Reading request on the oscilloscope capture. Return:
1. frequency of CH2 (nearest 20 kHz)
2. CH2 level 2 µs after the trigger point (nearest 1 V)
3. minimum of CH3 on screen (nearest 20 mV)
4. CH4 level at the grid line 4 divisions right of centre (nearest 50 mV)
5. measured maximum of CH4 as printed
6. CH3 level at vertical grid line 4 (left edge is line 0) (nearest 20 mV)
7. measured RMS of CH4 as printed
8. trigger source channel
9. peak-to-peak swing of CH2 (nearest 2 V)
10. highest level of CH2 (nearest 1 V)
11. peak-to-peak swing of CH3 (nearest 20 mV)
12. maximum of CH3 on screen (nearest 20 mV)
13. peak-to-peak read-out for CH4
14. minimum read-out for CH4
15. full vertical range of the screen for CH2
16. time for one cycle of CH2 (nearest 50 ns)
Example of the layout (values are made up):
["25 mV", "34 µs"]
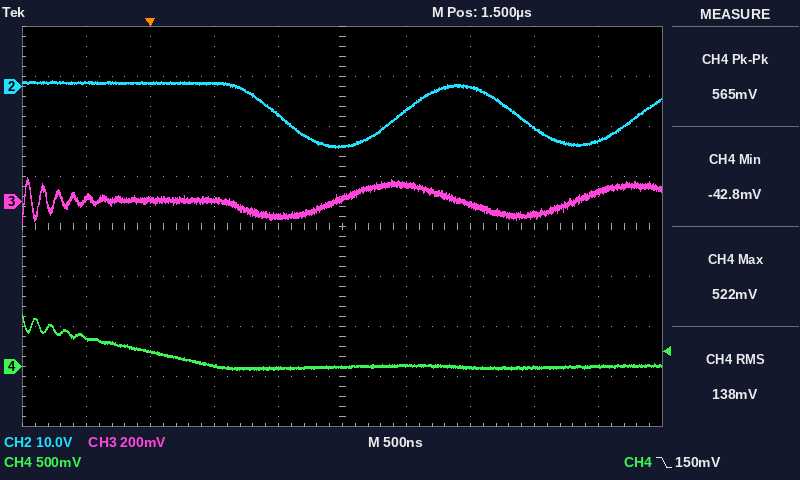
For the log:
["540 kHz", "-5 V", "-80 mV", "0 mV", "522 mV", "-60 mV", "138 mV", "CH4", "14 V", "1 V", "180 mV", "100 mV", "565 mV", "-42.8 mV", "80 V", "1.85 µs"]
